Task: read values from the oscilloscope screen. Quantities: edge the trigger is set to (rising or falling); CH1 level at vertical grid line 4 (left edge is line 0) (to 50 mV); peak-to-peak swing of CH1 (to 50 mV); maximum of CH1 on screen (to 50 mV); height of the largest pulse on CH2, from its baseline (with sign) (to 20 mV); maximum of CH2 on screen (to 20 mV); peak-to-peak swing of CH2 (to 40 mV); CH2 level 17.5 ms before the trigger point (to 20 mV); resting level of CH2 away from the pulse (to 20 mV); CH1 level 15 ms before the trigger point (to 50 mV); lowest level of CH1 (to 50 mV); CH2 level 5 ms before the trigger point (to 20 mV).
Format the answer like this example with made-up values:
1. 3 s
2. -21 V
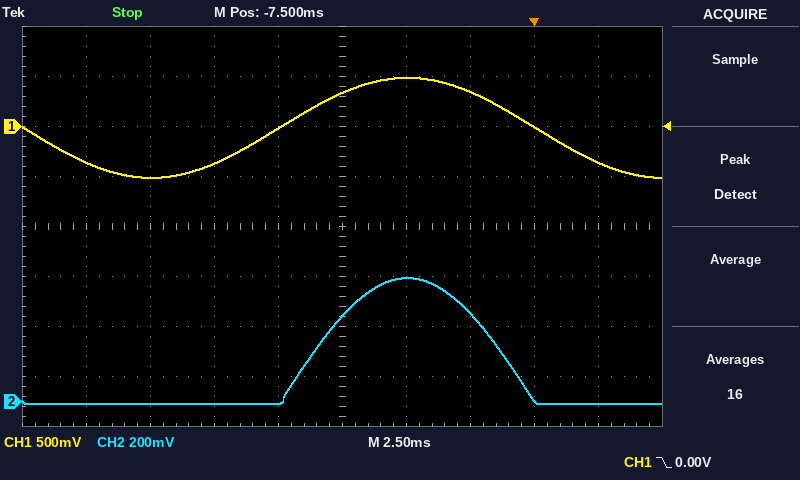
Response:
1. falling
2. 0 mV
3. 1.00 V
4. 500 mV
5. +500 mV
6. 500 mV
7. 520 mV
8. 0 mV
9. 0 mV
10. -500 mV
11. -500 mV
12. 500 mV
